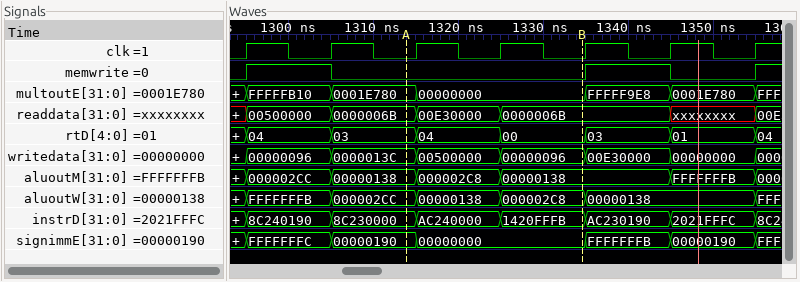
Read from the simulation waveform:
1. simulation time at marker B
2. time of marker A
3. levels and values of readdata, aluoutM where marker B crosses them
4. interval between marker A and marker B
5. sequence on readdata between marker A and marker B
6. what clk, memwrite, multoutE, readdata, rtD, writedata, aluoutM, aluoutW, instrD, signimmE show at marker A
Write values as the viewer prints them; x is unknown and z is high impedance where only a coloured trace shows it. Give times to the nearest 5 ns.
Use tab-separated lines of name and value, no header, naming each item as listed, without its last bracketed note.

simulation time at marker B	1335 ns
time of marker A	1315 ns
levels and values of readdata, aluoutM where marker B crosses them	readdata=0000006B, aluoutM=00000138
interval between marker A and marker B	20 ns
sequence on readdata between marker A and marker B	0000006B, 00E30000, 0000006B
what clk, memwrite, multoutE, readdata, rtD, writedata, aluoutM, aluoutW, instrD, signimmE show at marker A	clk=0, memwrite=0, multoutE=0001E780, readdata=0000006B, rtD=03, writedata=0000013C, aluoutM=00000138, aluoutW=000002CC, instrD=8C230000, signimmE=00000190
